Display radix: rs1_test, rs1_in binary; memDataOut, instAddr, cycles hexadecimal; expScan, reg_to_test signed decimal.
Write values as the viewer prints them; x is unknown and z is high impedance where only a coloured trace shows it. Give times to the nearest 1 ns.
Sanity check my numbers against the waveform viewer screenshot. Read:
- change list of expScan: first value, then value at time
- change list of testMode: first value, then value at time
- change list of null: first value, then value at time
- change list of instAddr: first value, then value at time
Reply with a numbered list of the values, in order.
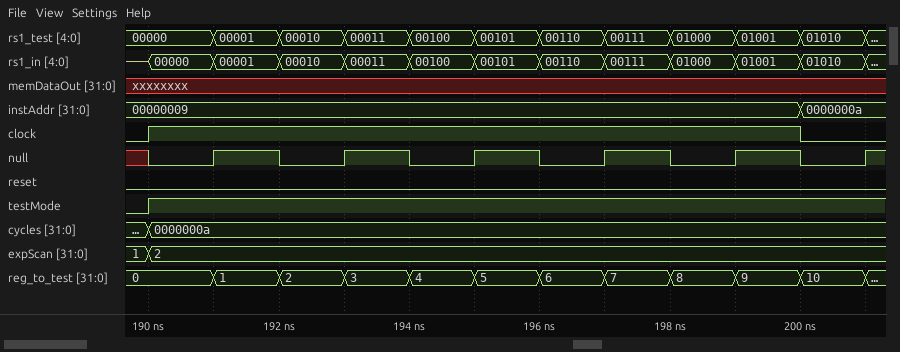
1. 1, 2 at 190 ns
2. 0, 1 at 190 ns
3. x, 0 at 190 ns, 1 at 191 ns, 0 at 192 ns, 1 at 193 ns, 0 at 194 ns, 1 at 195 ns, 0 at 196 ns, 1 at 197 ns, 0 at 198 ns, 1 at 199 ns, 0 at 200 ns, 1 at 201 ns
4. 00000009, 0000000a at 200 ns
